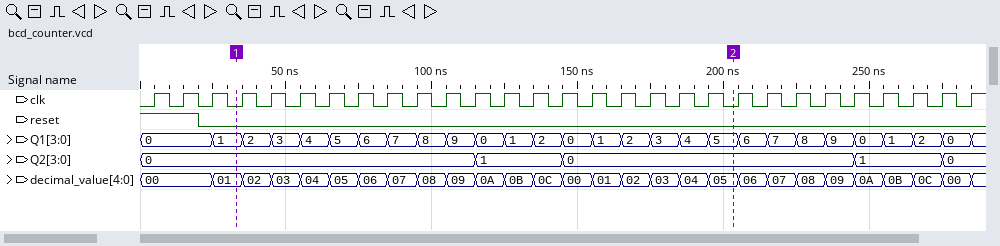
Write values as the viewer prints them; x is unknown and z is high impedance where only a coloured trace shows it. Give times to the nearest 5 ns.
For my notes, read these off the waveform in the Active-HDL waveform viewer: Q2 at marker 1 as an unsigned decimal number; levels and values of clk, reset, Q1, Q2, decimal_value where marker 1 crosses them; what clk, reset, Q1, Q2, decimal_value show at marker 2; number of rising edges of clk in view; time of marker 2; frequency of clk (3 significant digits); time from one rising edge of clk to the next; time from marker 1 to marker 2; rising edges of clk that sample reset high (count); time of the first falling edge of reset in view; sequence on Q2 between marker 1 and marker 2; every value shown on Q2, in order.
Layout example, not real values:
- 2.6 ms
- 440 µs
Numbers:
- 0
- clk=0, reset=0, Q1=1, Q2=0, decimal_value=01
- clk=0, reset=0, Q1=5, Q2=0, decimal_value=05
- 29
- 205 ns
- 100 MHz
- 10 ns
- 170 ns
- 2
- 20 ns
- 0, 1, 0
- 0, 1, 0, 1, 0
